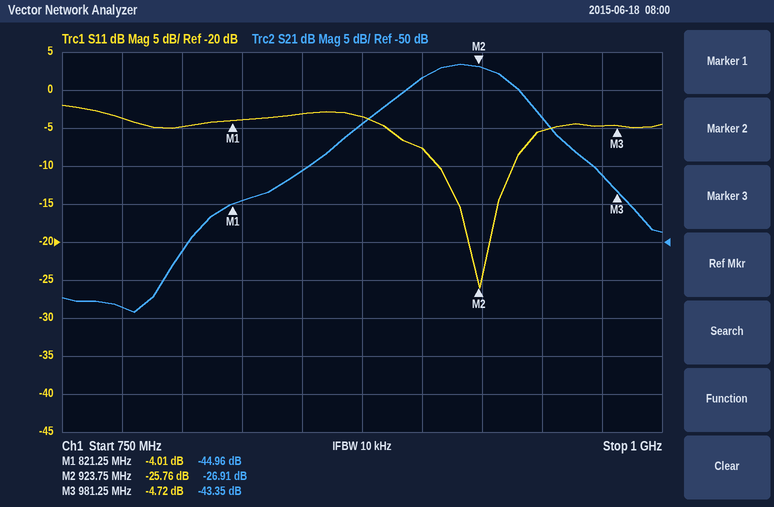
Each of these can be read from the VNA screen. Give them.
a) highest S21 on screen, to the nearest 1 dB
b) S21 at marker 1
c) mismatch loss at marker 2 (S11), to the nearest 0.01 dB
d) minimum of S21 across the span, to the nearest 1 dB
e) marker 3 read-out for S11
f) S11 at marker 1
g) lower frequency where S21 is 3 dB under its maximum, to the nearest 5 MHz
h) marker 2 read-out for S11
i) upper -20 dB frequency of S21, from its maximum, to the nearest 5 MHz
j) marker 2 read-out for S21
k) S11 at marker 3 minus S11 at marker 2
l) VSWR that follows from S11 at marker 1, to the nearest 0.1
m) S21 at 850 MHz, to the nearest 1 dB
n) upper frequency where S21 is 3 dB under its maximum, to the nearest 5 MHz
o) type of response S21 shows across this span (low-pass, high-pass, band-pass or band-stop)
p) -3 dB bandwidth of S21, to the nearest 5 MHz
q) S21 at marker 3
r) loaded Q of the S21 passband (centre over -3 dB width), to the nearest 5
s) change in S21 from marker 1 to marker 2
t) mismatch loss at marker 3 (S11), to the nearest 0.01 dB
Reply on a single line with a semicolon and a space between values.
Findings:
-27 dB; -44.96 dB; 0.01 dB; -59 dB; -4.72 dB; -4.01 dB; 895 MHz; -25.76 dB; 990 MHz; -26.91 dB; 21.04 dB; 4.4; -41 dB; 940 MHz; band-pass; 45 MHz; -43.35 dB; 20; 18.05 dB; 1.79 dB
